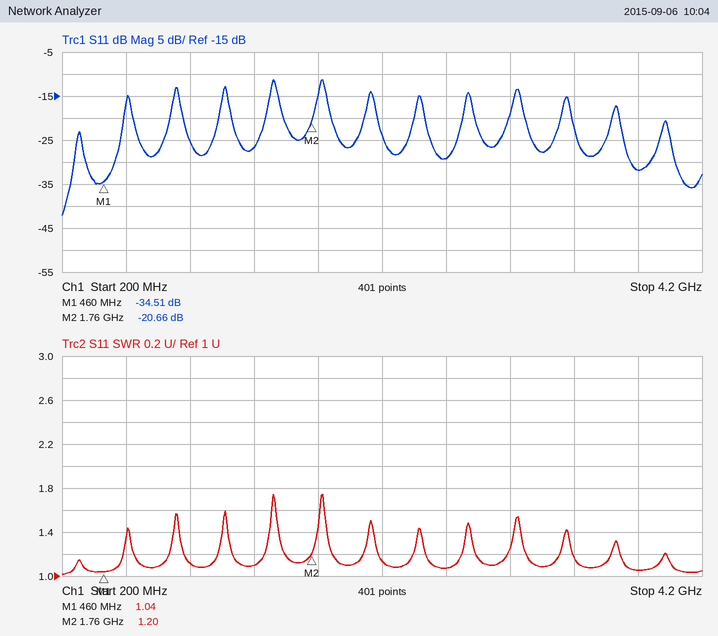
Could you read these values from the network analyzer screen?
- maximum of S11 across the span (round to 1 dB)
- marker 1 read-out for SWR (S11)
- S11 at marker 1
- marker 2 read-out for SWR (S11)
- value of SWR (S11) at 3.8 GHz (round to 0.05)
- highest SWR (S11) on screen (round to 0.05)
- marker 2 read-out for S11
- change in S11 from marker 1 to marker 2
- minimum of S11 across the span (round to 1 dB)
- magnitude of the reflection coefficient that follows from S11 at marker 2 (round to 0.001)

-11 dB
1.04
-34.51 dB
1.20
1.05
1.75
-20.66 dB
13.85 dB
-42 dB
0.093
